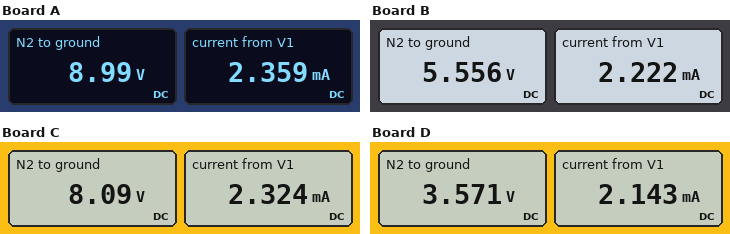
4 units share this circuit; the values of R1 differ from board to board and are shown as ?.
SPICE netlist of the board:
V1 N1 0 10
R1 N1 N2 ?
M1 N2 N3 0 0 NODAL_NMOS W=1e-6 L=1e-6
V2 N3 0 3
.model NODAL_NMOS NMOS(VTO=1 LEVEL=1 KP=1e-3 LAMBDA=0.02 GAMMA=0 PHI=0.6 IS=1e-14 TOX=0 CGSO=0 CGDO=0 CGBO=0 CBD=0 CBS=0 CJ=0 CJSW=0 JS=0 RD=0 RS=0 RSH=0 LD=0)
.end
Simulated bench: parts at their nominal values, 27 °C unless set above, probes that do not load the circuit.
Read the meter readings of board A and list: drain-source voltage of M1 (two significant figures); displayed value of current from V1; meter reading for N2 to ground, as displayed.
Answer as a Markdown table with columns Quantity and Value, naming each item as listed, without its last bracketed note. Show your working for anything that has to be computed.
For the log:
| Quantity | Value |
|---|---|
| drain-source voltage of M1 | 8.99 V = 9.0 V |
| displayed value of current from V1 | 2.359 mA |
| meter reading for N2 to ground, as displayed | 8.99 V |
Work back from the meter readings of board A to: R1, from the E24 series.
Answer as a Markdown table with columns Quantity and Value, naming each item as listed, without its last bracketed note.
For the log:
| Quantity | Value |
|---|---|
| R1, from the E24 series | 430 Ω |
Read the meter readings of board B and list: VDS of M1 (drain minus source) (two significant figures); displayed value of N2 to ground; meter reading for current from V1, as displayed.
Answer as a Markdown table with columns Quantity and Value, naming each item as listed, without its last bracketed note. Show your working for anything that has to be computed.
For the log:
| Quantity | Value |
|---|---|
| VDS of M1 (drain minus source) | 5.556 V = 5.6 V |
| displayed value of N2 to ground | 5.556 V |
| meter reading for current from V1, as displayed | 2.222 mA |
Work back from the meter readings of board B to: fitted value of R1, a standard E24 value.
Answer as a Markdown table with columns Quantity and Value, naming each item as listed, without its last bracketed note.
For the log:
| Quantity | Value |
|---|---|
| fitted value of R1, a standard E24 value | 2 kΩ |
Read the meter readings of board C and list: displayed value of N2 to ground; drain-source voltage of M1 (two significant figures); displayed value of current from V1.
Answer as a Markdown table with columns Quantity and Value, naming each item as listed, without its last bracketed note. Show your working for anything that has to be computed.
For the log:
| Quantity | Value |
|---|---|
| displayed value of N2 to ground | 8.09 V |
| drain-source voltage of M1 | 8.09 V = 8.1 V |
| displayed value of current from V1 | 2.324 mA |
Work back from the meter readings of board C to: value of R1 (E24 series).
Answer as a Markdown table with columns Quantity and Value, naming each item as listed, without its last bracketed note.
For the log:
| Quantity | Value |
|---|---|
| value of R1 | 820 Ω |
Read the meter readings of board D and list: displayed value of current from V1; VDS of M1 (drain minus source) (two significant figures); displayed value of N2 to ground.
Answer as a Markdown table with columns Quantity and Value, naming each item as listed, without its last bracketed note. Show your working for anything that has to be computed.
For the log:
| Quantity | Value |
|---|---|
| displayed value of current from V1 | 2.143 mA |
| VDS of M1 (drain minus source) | 3.571 V = 3.6 V |
| displayed value of N2 to ground | 3.571 V |
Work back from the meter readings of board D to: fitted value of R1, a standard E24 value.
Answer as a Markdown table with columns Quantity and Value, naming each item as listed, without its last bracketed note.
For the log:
| Quantity | Value |
|---|---|
| fitted value of R1, a standard E24 value | 3 kΩ |
